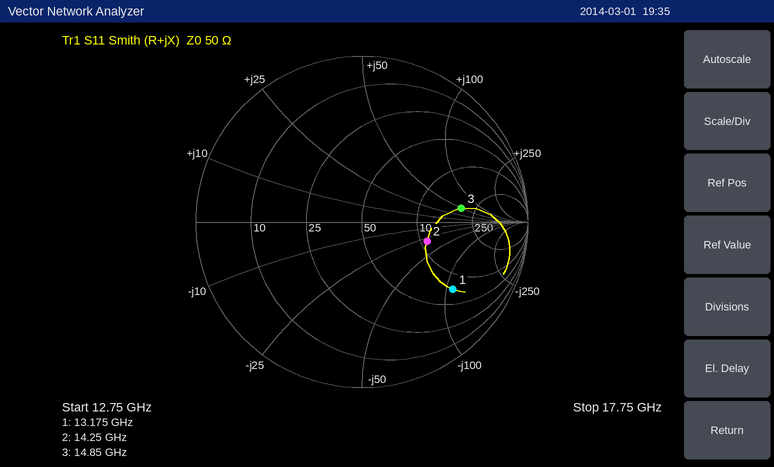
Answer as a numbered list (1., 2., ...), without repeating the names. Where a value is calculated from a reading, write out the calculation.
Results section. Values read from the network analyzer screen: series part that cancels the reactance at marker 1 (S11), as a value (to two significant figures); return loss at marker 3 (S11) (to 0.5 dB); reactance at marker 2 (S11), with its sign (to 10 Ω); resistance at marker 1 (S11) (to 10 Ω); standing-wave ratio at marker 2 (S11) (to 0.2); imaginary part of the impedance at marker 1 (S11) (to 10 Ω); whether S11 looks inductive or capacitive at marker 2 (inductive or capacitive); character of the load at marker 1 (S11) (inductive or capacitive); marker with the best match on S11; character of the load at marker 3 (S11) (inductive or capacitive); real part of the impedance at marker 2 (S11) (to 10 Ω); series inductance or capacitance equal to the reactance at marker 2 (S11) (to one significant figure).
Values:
1. L = 110 Ω/(2π × 13.175 GHz) ≈ 1.3 nH
2. 4.5 dB
3. -30 Ω
4. 70 Ω
5. 2.4
6. -110 Ω
7. capacitive
8. capacitive
9. marker 2
10. inductive
11. 110 Ω
12. C = 1/(2π × 14.25 GHz × 30 Ω) ≈ 372 fF, so 400 fF to one significant figure
